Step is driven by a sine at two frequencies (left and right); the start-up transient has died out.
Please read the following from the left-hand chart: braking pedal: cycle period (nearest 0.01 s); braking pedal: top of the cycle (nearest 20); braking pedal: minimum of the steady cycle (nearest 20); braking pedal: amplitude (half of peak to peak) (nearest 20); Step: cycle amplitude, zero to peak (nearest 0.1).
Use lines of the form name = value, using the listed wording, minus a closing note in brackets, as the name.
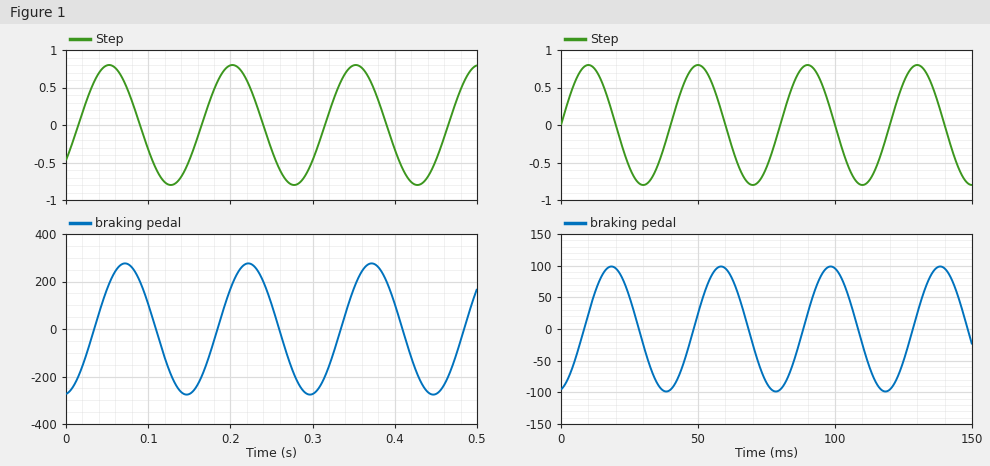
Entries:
braking pedal: cycle period = 0.15 s
braking pedal: top of the cycle = 280
braking pedal: minimum of the steady cycle = -280
braking pedal: amplitude (half of peak to peak) = 280
Step: cycle amplitude, zero to peak = 0.8
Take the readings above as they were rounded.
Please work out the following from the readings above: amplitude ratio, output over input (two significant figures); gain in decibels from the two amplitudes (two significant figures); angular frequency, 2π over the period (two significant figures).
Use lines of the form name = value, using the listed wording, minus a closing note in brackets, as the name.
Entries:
amplitude ratio, output over input = 350
gain in decibels from the two amplitudes = 51 dB
angular frequency, 2π over the period = 42 rad/s
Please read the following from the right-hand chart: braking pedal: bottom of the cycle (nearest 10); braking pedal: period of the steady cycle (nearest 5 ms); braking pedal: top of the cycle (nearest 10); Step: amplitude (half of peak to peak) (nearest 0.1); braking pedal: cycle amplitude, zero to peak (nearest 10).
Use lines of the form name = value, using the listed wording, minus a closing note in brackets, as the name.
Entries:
braking pedal: bottom of the cycle = -100
braking pedal: period of the steady cycle = 40 ms
braking pedal: top of the cycle = 100
Step: amplitude (half of peak to peak) = 0.8
braking pedal: cycle amplitude, zero to peak = 100
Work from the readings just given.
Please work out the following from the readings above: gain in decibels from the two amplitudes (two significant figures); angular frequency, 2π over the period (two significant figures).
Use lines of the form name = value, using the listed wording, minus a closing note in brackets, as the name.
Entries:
gain in decibels from the two amplitudes = 42 dB
angular frequency, 2π over the period = 0.16 rad/ms
